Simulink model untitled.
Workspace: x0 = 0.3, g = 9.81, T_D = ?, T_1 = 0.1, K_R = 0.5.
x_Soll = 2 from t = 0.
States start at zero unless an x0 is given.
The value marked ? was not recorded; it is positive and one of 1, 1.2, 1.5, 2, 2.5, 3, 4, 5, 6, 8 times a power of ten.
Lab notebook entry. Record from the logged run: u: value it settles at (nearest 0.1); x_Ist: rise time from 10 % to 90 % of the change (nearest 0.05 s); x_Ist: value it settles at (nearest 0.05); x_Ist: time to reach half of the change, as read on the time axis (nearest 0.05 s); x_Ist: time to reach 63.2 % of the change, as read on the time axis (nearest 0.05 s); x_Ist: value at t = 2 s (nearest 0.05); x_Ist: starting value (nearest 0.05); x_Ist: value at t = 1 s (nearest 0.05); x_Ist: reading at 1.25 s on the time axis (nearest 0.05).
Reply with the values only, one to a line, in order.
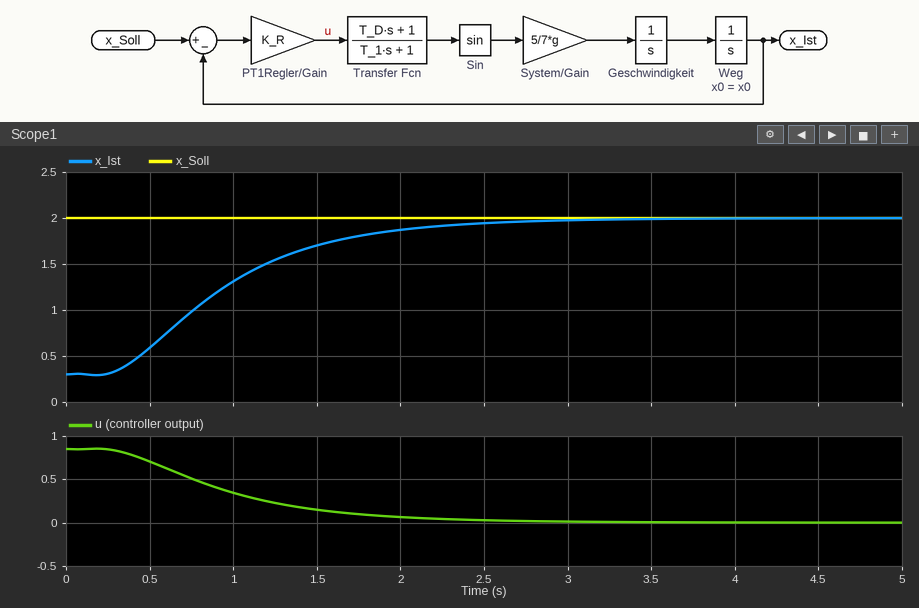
0.0
1.40 s
2.00
0.85 s
1.05 s
1.85
0.30
1.30
1.55
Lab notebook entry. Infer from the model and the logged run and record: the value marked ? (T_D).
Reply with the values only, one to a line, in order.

1
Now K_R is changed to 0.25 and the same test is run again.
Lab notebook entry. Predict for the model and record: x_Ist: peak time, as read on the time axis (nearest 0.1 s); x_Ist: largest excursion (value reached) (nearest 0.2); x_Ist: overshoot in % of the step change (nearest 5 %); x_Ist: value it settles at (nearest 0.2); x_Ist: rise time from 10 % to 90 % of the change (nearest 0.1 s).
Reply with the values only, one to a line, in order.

2.5 s
2.2
10 %
2.0
1.1 s
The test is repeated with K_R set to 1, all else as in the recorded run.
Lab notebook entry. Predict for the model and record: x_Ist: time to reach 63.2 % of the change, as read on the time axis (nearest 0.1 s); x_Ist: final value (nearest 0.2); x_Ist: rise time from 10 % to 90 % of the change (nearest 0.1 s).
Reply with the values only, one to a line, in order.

1.3 s
2.0
1.8 s
